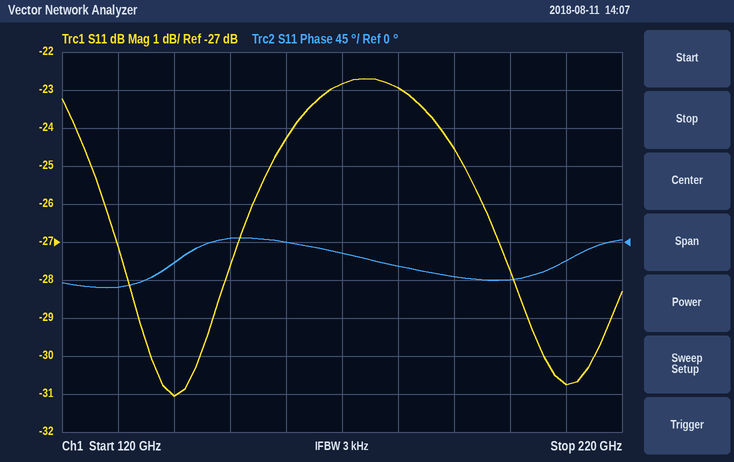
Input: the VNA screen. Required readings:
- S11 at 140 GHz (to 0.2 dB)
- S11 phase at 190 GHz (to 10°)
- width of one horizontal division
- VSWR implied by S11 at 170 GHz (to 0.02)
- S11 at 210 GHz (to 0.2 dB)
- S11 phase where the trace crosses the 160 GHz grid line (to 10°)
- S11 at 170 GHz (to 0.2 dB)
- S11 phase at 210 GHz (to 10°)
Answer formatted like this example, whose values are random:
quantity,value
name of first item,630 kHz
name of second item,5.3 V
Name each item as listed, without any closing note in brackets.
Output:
quantity,value
S11 at 140 GHz,-31.0 dB
S11 phase at 190 GHz,-40°
width of one horizontal division,10 GHz
VSWR implied by S11 at 170 GHz,1.16
S11 at 210 GHz,-30.8 dB
S11 phase where the trace crosses the 160 GHz grid line,0°
S11 at 170 GHz,-22.8 dB
S11 phase at 210 GHz,-20°
